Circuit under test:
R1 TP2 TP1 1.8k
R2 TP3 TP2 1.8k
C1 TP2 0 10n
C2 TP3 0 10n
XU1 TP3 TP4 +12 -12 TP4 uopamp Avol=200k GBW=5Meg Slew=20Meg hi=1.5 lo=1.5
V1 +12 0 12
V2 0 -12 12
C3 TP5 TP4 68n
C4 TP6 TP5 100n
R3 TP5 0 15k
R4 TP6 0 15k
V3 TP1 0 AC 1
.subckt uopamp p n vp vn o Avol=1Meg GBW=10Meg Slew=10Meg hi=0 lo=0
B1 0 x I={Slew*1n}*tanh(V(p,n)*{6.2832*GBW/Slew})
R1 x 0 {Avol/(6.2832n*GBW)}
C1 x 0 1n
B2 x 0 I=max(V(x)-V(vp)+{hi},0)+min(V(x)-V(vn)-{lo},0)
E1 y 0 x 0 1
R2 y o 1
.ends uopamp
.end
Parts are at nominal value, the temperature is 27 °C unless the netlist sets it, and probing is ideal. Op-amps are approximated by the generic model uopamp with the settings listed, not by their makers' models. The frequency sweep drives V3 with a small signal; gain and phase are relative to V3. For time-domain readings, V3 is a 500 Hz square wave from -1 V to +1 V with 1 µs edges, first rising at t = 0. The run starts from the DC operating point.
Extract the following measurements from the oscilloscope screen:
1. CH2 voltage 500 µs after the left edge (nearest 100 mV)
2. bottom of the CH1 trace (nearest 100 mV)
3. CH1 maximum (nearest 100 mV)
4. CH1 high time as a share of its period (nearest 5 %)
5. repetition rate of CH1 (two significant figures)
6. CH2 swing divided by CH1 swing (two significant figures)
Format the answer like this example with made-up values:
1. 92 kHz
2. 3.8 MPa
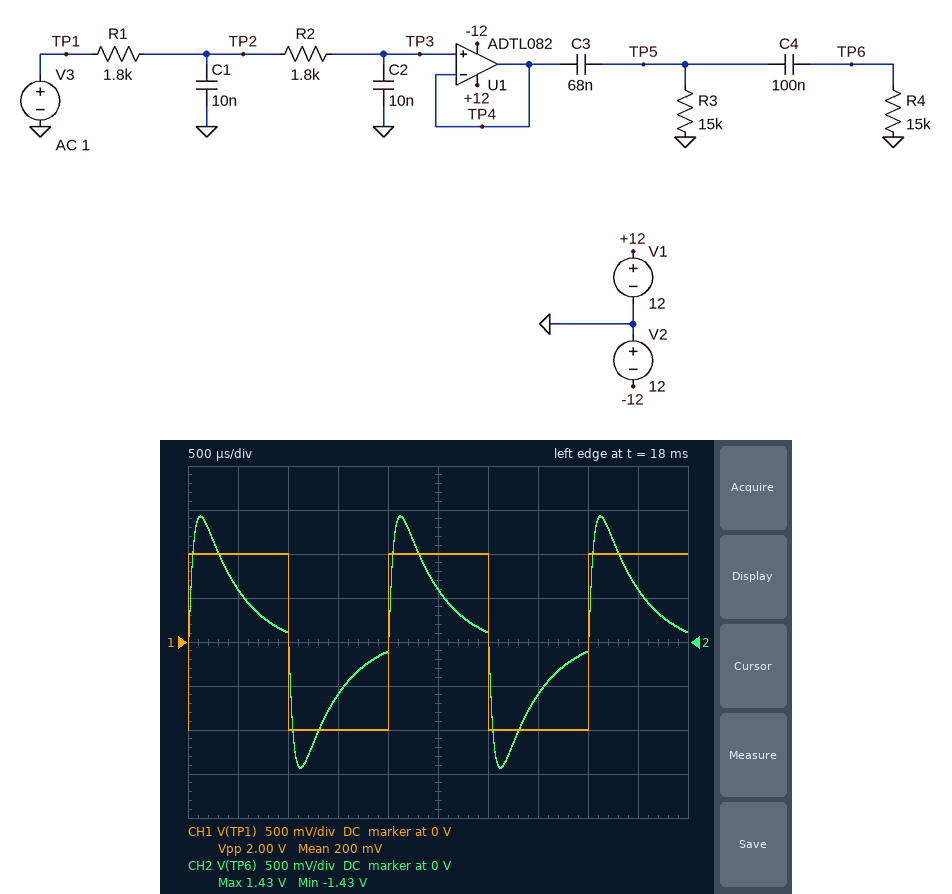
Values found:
1. 600 mV
2. -1.0 V
3. 1.0 V
4. 50 %
5. 500 Hz
6. 1.4
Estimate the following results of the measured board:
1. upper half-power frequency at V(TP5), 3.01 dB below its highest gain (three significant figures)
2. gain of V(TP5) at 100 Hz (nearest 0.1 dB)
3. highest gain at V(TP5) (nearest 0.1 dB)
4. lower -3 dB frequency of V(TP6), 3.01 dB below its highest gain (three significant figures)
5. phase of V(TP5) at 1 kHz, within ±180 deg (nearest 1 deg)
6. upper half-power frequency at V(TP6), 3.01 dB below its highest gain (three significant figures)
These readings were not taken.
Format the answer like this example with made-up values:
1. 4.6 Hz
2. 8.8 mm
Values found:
1. 3.95 kHz
2. -9.3 dB
3. -0.9 dB
4. 315 Hz
5. -2 deg
6. 3.97 kHz
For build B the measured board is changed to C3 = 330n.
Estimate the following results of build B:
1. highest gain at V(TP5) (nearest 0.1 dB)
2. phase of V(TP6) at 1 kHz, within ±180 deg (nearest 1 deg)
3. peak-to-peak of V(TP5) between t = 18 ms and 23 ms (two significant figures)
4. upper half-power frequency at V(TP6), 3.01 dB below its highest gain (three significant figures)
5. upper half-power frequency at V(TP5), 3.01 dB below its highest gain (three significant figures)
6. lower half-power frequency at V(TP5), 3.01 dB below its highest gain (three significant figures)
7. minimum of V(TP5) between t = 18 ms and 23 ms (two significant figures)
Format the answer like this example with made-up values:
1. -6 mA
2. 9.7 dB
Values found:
1. -0.3 dB
2. -9 deg
3. 2.2 V
4. 3.59 kHz
5. 3.50 kHz
6. 50.5 Hz
7. -1.1 V
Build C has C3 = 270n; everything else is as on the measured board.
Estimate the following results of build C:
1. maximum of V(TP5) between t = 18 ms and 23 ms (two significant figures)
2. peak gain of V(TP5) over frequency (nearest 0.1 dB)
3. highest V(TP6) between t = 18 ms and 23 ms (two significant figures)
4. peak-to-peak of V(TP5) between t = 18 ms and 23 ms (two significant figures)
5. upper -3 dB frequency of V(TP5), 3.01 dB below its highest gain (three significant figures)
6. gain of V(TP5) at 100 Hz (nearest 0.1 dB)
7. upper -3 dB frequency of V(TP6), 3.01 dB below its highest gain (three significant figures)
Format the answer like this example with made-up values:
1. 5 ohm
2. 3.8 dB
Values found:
1. 1.1 V
2. -0.3 dB
3. 1.3 V
4. 2.2 V
5. 3.53 kHz
6. -2.5 dB
7. 3.61 kHz
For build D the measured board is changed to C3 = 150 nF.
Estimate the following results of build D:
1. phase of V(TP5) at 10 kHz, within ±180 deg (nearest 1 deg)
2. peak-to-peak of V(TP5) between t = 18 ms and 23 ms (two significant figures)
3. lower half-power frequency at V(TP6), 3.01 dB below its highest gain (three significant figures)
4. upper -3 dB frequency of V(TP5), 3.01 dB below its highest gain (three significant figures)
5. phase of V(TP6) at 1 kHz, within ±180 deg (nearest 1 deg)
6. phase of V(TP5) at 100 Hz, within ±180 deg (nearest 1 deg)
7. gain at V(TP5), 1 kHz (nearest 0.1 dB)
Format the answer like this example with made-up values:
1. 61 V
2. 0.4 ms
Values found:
1. -94 deg
2. 2.4 V
3. 195 Hz
4. 3.65 kHz
5. -5 deg
6. 36 deg
7. -0.5 dB
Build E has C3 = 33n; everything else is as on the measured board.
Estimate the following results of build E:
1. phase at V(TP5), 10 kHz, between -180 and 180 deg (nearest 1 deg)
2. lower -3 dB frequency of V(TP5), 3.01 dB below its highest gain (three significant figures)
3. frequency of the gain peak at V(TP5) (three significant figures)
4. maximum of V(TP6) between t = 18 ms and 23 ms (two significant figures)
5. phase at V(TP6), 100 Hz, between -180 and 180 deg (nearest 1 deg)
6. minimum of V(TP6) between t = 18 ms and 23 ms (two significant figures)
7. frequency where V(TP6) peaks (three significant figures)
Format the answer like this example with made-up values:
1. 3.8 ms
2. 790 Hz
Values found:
1. -91 deg
2. 501 Hz
3. 1.52 kHz
4. 1.3 V
5. 106 deg
6. -1.3 V
7. 1.53 kHz
